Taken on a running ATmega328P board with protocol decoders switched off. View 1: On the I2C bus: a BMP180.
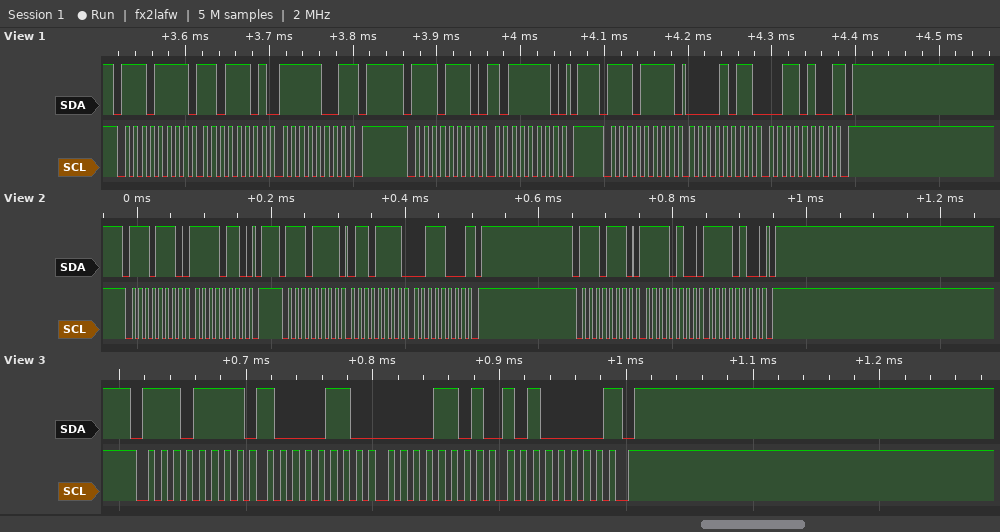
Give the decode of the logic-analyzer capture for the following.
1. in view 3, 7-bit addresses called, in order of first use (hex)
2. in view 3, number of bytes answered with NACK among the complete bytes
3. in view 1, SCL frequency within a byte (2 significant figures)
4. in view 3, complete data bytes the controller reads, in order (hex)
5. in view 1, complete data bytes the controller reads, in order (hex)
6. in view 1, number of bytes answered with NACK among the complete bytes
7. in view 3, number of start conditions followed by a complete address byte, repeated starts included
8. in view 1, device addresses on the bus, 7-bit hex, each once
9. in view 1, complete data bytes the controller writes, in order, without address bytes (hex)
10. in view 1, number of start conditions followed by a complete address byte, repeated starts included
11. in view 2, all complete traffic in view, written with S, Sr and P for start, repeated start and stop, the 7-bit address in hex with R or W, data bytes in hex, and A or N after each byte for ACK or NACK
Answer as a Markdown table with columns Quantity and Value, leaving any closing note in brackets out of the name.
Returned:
| Quantity | Value |
|---|---|
| in view 3, 7-bit addresses called, in order of first use | 0x77 |
| in view 3, number of bytes answered with NACK among the complete bytes | 1 |
| in view 1, SCL frequency within a byte | 100 kHz |
| in view 3, complete data bytes the controller reads, in order | 86 0D A0 |
| in view 1, complete data bytes the controller reads, in order | DD F9 0B 34 |
| in view 1, number of bytes answered with NACK among the complete bytes | 2 |
| in view 3, number of start conditions followed by a complete address byte, repeated starts included | 1 |
| in view 1, device addresses on the bus, 7-bit hex, each once | 0x77 |
| in view 1, complete data bytes the controller writes, in order, without address bytes | BE |
| in view 1, number of start conditions followed by a complete address byte, repeated starts included | 3 |
| in view 2, all complete traffic in view, written with S, Sr and P for start, repeated start and stop, the 7-bit address in hex with R or W, data bytes in hex, and A or N after each byte for ACK or NACK | S 77W A F6 A P S 77R A 6F A 38 N P S 77W A F4 A F4 A P |
